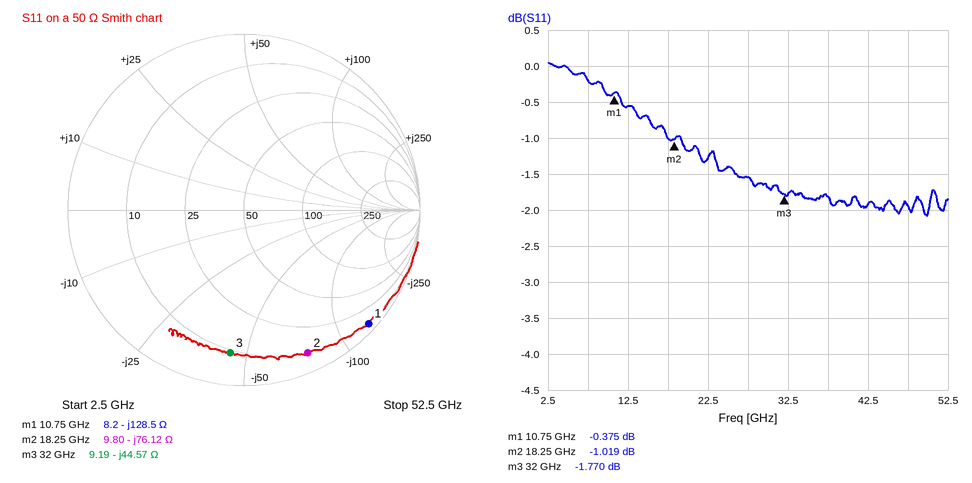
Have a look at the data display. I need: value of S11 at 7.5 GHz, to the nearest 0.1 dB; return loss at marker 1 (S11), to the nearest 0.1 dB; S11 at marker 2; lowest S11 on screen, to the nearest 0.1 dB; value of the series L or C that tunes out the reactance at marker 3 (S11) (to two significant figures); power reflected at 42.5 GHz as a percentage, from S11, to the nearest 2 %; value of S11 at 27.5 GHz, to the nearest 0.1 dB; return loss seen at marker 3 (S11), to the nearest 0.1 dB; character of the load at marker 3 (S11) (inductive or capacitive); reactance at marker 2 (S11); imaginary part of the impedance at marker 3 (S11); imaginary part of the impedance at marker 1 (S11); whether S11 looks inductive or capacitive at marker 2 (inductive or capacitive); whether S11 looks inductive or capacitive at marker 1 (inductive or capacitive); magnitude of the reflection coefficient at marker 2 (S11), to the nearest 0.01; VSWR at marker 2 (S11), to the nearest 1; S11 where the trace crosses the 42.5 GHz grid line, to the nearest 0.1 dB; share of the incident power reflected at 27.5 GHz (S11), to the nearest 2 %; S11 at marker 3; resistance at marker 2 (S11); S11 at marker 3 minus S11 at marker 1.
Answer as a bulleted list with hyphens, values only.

- -0.2 dB
- 0.4 dB
- -1.019 dB
- -2.1 dB
- 220 pH
- 64 %
- -1.5 dB
- 1.8 dB
- capacitive
- -76.12 Ω
- -44.57 Ω
- -128.5 Ω
- capacitive
- capacitive
- 0.89
- 17
- -1.9 dB
- 70 %
- -1.770 dB
- 9.80 Ω
- -1.395 dB
